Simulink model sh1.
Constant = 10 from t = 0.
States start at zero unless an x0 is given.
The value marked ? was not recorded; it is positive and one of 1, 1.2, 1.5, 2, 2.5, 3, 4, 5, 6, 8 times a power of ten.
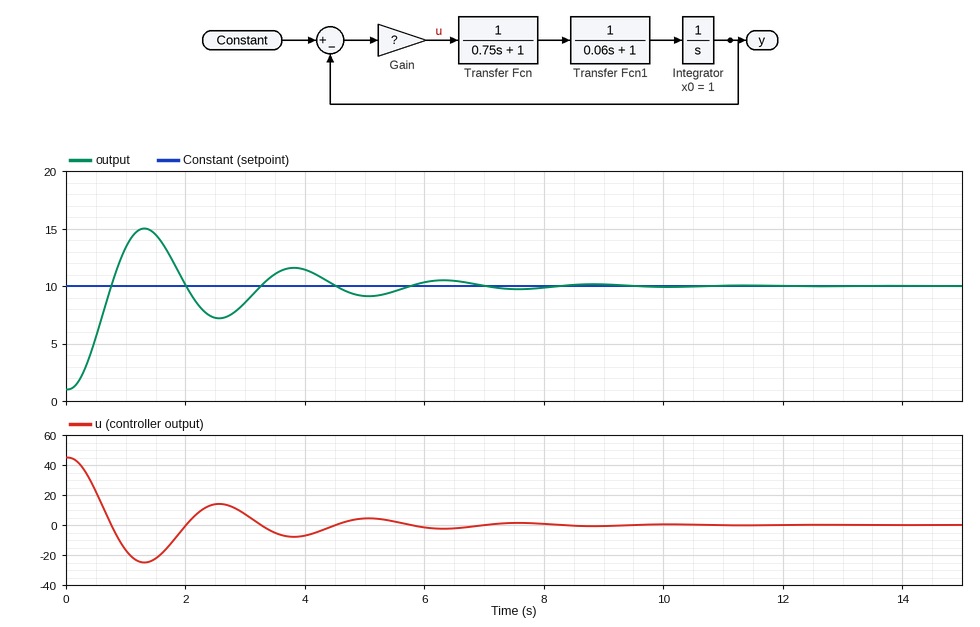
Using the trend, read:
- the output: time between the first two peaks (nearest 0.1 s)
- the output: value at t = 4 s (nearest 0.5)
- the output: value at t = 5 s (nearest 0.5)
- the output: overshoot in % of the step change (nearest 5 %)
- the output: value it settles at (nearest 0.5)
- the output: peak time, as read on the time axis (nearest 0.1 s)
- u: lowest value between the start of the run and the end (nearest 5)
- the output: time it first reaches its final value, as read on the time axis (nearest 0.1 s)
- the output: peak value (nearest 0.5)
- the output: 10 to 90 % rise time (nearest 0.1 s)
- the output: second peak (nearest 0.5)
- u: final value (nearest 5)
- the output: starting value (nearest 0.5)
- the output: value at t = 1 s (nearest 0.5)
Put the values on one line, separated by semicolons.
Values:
2.5 s; 11.5; 9.0; 55 %; 10.0; 1.3 s; -25; 0.8 s; 15.0; 0.5 s; 11.5; 0; 1.0; 13.5
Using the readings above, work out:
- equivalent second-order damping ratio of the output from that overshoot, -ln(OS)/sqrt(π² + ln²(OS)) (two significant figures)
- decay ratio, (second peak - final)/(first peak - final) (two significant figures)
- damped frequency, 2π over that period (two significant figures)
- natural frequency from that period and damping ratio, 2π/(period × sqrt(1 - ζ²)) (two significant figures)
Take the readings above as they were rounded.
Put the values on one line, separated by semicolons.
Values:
0.19; 0.30; 2.5 rad/s; 2.6 rad/s
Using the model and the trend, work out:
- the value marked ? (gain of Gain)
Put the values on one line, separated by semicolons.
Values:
5
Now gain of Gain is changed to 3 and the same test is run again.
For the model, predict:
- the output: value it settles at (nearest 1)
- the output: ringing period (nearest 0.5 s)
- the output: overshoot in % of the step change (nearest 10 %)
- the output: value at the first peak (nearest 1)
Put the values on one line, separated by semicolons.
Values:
10; 3.5 s; 40 %; 14
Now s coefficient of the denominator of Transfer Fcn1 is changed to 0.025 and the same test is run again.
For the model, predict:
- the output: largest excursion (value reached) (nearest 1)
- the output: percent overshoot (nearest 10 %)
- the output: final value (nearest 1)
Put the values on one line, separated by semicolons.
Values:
14; 50 %; 10
